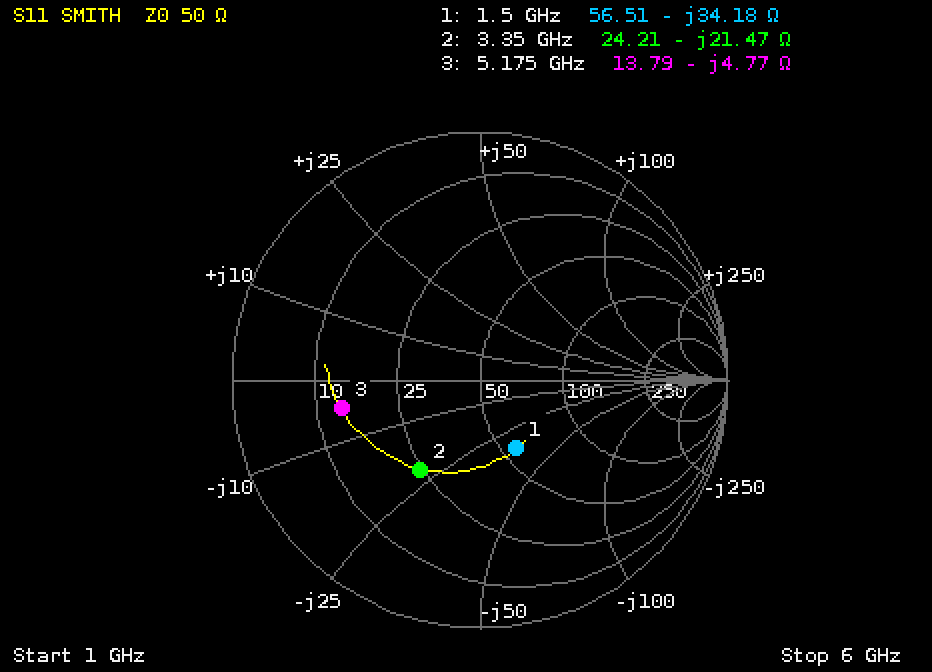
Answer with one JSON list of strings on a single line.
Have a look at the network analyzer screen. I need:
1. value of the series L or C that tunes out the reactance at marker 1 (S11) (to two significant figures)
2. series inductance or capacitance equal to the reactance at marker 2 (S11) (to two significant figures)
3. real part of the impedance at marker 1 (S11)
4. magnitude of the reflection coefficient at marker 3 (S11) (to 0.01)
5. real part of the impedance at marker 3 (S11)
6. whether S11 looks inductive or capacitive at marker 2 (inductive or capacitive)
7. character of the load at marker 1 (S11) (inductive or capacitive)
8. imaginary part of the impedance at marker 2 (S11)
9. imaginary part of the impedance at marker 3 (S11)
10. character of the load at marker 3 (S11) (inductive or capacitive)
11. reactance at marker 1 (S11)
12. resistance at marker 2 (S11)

["3.6 nH", "2.2 pF", "56.51 Ω", "0.57", "13.79 Ω", "capacitive", "capacitive", "-21.47 Ω", "-4.77 Ω", "capacitive", "-34.18 Ω", "24.21 Ω"]
